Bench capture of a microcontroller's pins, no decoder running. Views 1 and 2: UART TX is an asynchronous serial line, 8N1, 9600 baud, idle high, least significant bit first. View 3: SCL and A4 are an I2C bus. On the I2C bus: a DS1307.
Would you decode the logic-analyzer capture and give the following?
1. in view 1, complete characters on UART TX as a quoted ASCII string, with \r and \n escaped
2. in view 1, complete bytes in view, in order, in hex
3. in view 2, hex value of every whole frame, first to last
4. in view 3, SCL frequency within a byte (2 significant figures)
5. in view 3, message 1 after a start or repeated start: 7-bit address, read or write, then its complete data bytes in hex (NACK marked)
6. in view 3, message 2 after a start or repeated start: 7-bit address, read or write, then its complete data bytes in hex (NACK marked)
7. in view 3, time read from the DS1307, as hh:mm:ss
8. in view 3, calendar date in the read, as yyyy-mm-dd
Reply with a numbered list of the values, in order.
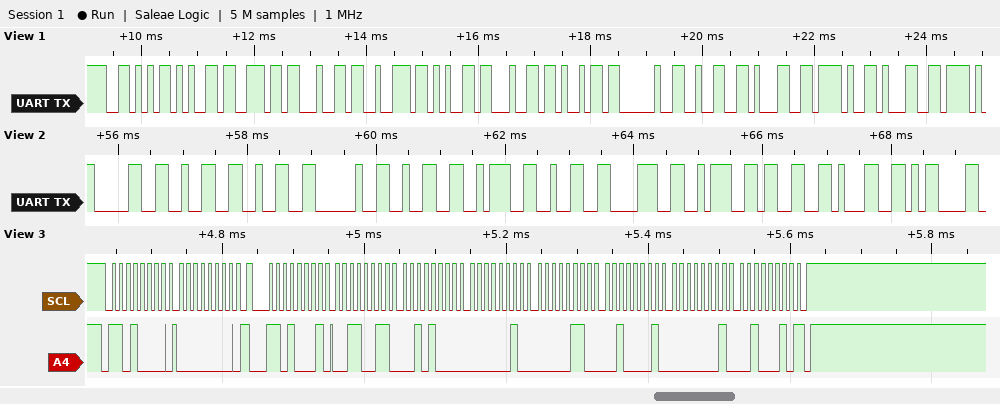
1. "Vendredi 21/1"
2. 56 65 6E 64 72 65 64 69 20 32 31 2F 31
3. 30 32 32 20 32 3A 32 38 3A 33 31 0D
4. 100 kHz
5. 0x68 write: 00
6. 0x68 read: 33 28 02 06 21 01 22 NACK
7. 02:28:33
8. 2022-01-21
